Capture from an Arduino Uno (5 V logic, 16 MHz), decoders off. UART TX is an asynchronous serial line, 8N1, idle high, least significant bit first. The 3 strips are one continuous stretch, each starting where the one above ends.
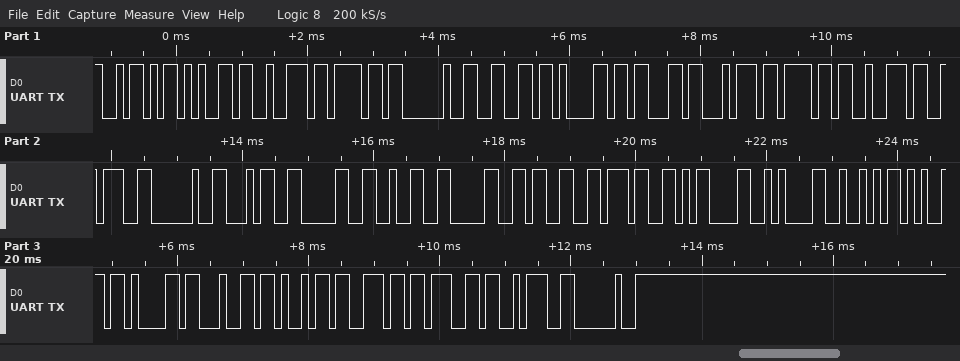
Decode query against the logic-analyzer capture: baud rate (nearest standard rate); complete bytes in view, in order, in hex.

9600 baud
5A 65 72 6F 20 66 61 63 74 6F 72 3A 20 34 30 32 30 33 37 0D 0A 52 65 61 64 69 6E 67 3A 20
